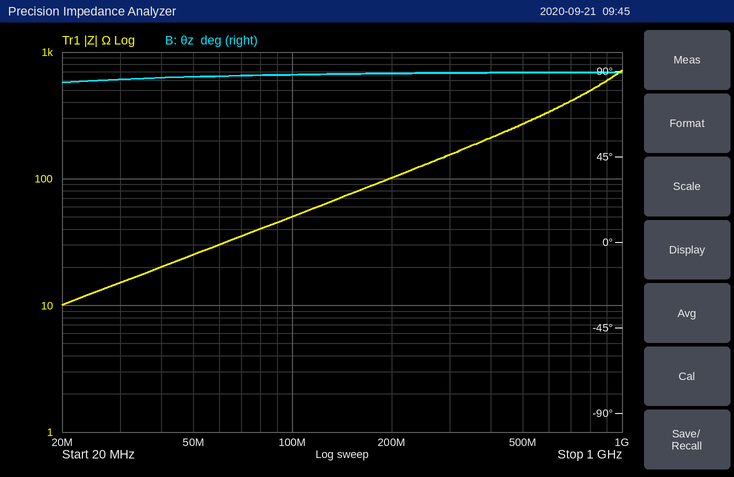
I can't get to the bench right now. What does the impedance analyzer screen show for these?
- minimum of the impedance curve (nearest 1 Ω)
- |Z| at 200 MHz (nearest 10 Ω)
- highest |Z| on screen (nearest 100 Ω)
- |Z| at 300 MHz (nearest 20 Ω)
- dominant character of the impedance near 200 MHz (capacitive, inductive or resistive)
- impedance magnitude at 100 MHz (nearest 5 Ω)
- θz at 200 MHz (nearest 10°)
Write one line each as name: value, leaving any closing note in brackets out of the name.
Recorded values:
minimum of the impedance curve: 10 Ω
|Z| at 200 MHz: 100 Ω
highest |Z| on screen: 700 Ω
|Z| at 300 MHz: 160 Ω
dominant character of the impedance near 200 MHz: inductive
impedance magnitude at 100 MHz: 50 Ω
θz at 200 MHz: 90°
